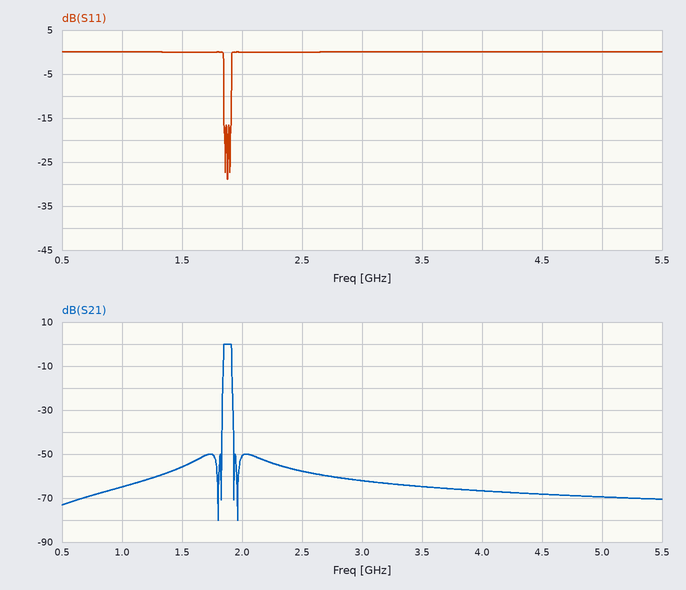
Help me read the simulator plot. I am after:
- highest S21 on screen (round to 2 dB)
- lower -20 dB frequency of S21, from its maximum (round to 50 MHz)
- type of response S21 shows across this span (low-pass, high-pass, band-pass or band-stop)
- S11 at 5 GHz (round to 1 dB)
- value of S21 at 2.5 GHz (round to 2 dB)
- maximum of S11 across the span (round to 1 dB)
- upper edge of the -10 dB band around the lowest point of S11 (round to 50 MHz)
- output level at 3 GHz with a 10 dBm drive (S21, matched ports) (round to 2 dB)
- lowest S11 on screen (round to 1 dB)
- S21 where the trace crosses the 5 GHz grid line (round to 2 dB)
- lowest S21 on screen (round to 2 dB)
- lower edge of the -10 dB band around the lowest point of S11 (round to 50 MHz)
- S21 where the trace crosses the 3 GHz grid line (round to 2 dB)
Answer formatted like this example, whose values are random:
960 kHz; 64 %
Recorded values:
0 dB; 1.85 GHz; band-pass; 0 dB; -58 dB; 0 dB; 1.90 GHz; -52 dBm; -29 dB; -70 dB; -80 dB; 1.85 GHz; -62 dB
